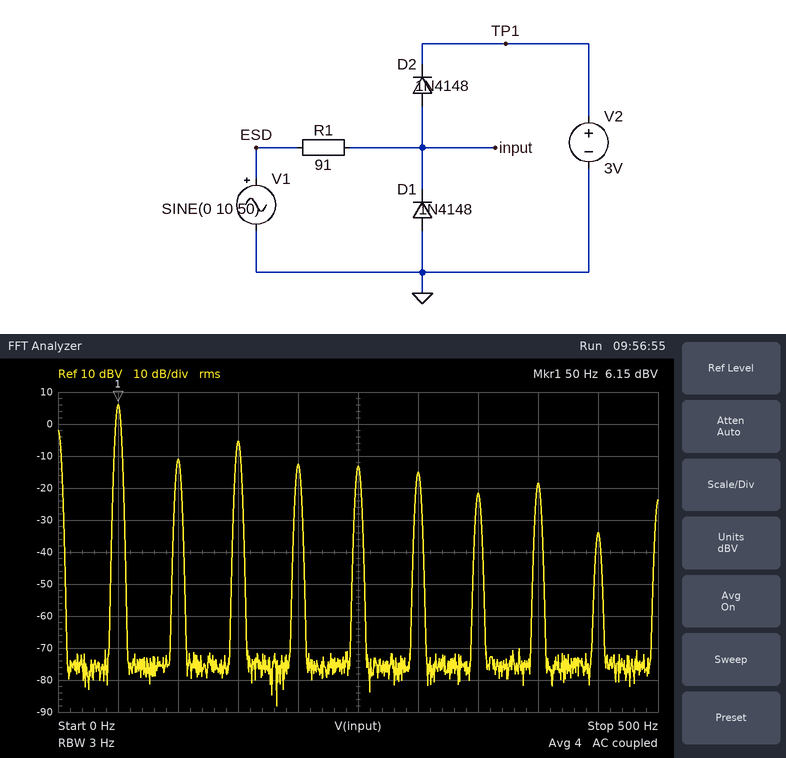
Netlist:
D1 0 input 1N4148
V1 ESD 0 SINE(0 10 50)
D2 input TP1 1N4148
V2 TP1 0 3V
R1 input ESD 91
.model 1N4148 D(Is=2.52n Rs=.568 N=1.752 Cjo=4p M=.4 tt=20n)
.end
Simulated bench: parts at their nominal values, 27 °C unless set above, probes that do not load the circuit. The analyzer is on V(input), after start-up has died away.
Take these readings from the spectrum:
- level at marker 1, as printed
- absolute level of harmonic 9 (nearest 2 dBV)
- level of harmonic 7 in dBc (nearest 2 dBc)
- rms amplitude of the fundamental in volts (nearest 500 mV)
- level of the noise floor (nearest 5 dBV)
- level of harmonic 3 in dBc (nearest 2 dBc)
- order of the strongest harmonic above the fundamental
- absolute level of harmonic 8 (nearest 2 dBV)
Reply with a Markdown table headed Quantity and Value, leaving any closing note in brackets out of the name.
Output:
| Quantity | Value |
|---|---|
| level at marker 1, as printed | 6.15 dBV |
| absolute level of harmonic 9 | -34 dBV |
| level of harmonic 7 in dBc | -28 dBc |
| rms amplitude of the fundamental in volts | 2.0 V |
| level of the noise floor | -75 dBV |
| level of harmonic 3 in dBc | -12 dBc |
| order of the strongest harmonic above the fundamental | 3 |
| absolute level of harmonic 8 | -18 dBV |
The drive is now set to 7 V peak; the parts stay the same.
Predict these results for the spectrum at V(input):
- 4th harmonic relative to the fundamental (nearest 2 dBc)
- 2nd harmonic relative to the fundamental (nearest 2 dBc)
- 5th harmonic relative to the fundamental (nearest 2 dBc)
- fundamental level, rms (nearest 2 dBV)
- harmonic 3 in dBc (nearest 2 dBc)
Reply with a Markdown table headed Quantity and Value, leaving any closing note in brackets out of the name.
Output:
| Quantity | Value |
|---|---|
| 4th harmonic relative to the fundamental | -18 dBc |
| 2nd harmonic relative to the fundamental | -14 dBc |
| 5th harmonic relative to the fundamental | -26 dBc |
| fundamental level, rms | 6 dBV |
| harmonic 3 in dBc | -14 dBc |
